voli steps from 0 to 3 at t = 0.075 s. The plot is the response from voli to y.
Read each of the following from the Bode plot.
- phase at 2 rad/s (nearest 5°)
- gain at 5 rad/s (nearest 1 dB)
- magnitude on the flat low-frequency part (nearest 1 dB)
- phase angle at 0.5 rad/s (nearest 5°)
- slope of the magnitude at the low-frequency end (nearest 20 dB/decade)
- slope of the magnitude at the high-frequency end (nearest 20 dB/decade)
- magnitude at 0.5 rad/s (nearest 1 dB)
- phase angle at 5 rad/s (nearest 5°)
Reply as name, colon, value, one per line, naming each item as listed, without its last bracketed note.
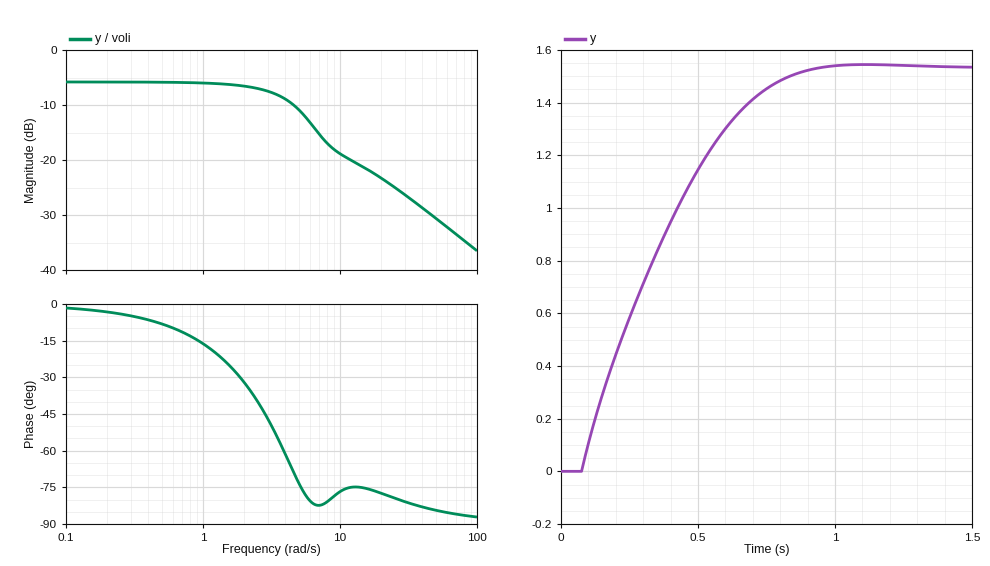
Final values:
phase at 2 rad/s: -30°
gain at 5 rad/s: -11 dB
magnitude on the flat low-frequency part: -6 dB
phase angle at 0.5 rad/s: -10°
slope of the magnitude at the low-frequency end: 0 dB/decade
slope of the magnitude at the high-frequency end: -20 dB/decade
magnitude at 0.5 rad/s: -6 dB
phase angle at 5 rad/s: -75°
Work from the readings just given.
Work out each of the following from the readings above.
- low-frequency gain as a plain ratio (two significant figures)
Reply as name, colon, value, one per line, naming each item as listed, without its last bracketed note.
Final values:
low-frequency gain as a plain ratio: 0.50
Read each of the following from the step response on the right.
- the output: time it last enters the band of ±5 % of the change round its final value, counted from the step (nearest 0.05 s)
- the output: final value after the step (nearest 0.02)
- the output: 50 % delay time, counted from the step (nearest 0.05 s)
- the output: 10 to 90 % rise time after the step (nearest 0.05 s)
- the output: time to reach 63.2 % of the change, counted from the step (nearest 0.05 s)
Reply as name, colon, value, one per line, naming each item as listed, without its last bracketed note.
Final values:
the output: time it last enters the band of ±5 % of the change round its final value, counted from the step: 0.70 s
the output: final value after the step: 1.54
the output: 50 % delay time, counted from the step: 0.25 s
the output: 10 to 90 % rise time after the step: 0.55 s
the output: time to reach 63.2 % of the change, counted from the step: 0.35 s
